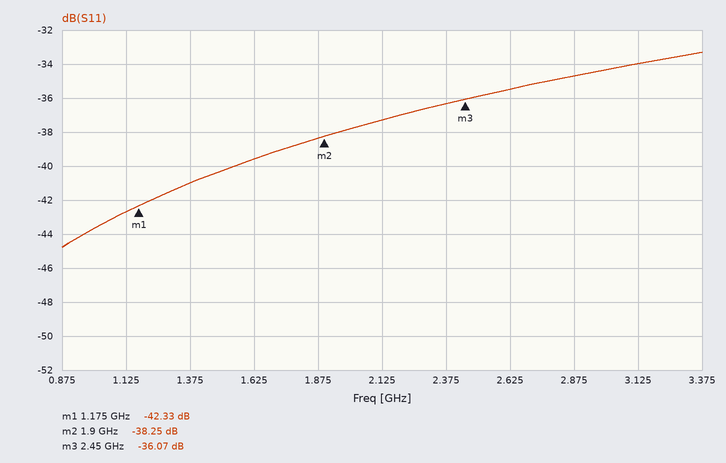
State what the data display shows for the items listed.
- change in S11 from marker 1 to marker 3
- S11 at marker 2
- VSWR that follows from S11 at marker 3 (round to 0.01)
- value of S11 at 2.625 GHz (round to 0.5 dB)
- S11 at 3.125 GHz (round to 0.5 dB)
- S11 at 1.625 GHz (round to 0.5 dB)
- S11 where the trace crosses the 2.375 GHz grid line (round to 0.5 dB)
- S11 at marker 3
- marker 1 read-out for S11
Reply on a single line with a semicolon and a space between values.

6.26 dB; -38.25 dB; 1.03; -35.5 dB; -34.0 dB; -39.5 dB; -36.5 dB; -36.07 dB; -42.33 dB
